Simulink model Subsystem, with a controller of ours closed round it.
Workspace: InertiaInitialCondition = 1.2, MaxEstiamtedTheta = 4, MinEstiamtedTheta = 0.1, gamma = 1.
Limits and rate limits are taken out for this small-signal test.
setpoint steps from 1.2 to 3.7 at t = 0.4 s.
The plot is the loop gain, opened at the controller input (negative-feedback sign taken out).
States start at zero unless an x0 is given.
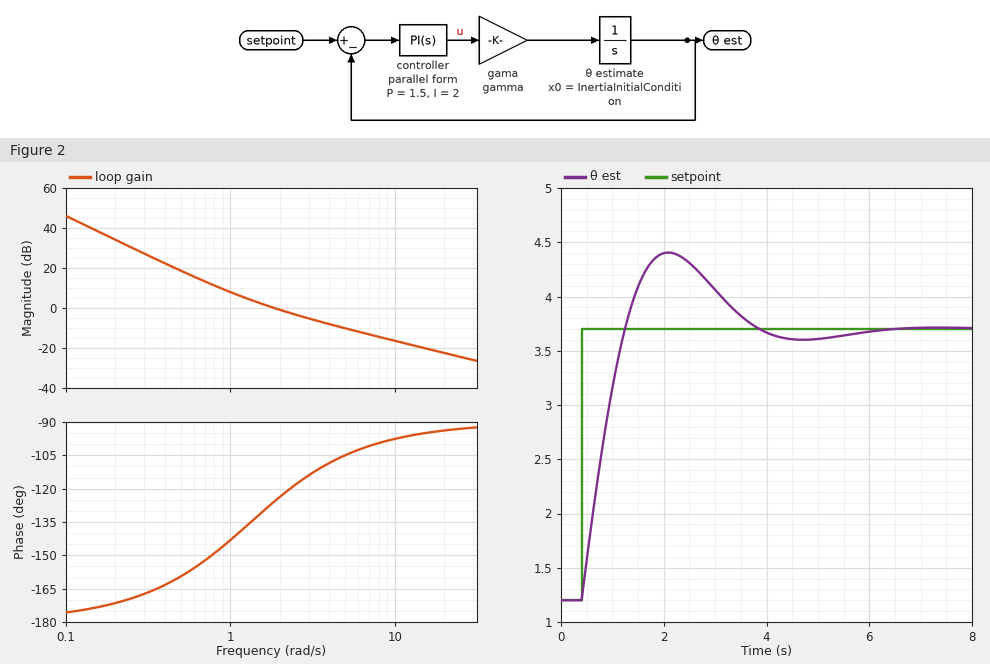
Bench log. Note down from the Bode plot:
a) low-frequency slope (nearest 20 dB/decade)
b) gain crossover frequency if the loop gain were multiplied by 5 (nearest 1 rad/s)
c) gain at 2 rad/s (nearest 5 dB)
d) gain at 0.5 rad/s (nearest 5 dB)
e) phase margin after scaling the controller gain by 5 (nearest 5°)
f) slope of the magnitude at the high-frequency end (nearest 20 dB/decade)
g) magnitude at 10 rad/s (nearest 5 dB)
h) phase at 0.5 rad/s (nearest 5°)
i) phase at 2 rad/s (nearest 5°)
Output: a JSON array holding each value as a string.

["-40 dB/decade", "8 rad/s", "0 dB", "20 dB", "80°", "-20 dB/decade", "-15 dB", "-160°", "-125°"]
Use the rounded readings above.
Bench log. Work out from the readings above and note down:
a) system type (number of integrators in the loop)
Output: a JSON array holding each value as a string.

["2"]
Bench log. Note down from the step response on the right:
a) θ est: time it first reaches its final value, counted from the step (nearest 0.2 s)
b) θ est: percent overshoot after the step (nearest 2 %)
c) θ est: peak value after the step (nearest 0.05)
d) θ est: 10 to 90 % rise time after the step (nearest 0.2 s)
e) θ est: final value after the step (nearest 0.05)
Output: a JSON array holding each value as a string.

["0.8 s", "28 %", "4.40", "0.6 s", "3.70"]
